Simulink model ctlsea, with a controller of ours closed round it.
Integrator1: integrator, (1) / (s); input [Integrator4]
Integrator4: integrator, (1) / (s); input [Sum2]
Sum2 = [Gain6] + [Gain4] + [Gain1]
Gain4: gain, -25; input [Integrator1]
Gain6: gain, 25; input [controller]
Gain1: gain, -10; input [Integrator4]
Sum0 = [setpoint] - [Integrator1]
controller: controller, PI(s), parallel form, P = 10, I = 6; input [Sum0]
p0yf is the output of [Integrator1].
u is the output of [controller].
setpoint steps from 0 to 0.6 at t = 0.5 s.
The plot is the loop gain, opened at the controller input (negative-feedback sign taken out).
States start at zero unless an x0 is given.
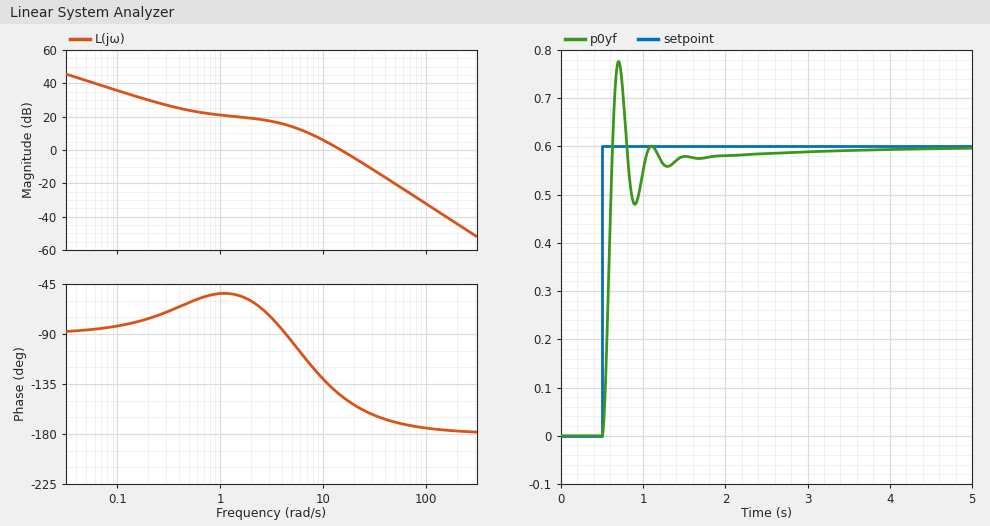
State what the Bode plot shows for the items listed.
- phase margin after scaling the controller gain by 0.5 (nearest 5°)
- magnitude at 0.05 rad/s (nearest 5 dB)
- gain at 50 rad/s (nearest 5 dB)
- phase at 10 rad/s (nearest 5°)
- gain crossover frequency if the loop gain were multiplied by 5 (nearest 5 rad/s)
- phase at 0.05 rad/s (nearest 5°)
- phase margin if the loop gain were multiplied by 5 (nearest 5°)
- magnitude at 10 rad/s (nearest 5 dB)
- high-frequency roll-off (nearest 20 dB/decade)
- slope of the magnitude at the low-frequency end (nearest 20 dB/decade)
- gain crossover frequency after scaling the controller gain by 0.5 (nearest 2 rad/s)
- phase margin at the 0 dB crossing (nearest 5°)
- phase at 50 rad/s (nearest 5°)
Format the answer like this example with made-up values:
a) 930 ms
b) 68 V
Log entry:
a) 50°
b) 40 dB
c) -20 dB
d) -130°
e) 35 rad/s
f) -85°
g) 15°
h) 5 dB
i) -40 dB/decade
j) -20 dB/decade
k) 10 rad/s
l) 35°
m) -170°
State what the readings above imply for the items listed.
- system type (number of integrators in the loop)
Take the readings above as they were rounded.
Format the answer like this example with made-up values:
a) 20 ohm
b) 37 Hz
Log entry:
a) 1
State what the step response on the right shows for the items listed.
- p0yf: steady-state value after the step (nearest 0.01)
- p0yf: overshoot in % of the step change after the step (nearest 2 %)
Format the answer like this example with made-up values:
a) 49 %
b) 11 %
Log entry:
a) 0.60
b) 30 %
